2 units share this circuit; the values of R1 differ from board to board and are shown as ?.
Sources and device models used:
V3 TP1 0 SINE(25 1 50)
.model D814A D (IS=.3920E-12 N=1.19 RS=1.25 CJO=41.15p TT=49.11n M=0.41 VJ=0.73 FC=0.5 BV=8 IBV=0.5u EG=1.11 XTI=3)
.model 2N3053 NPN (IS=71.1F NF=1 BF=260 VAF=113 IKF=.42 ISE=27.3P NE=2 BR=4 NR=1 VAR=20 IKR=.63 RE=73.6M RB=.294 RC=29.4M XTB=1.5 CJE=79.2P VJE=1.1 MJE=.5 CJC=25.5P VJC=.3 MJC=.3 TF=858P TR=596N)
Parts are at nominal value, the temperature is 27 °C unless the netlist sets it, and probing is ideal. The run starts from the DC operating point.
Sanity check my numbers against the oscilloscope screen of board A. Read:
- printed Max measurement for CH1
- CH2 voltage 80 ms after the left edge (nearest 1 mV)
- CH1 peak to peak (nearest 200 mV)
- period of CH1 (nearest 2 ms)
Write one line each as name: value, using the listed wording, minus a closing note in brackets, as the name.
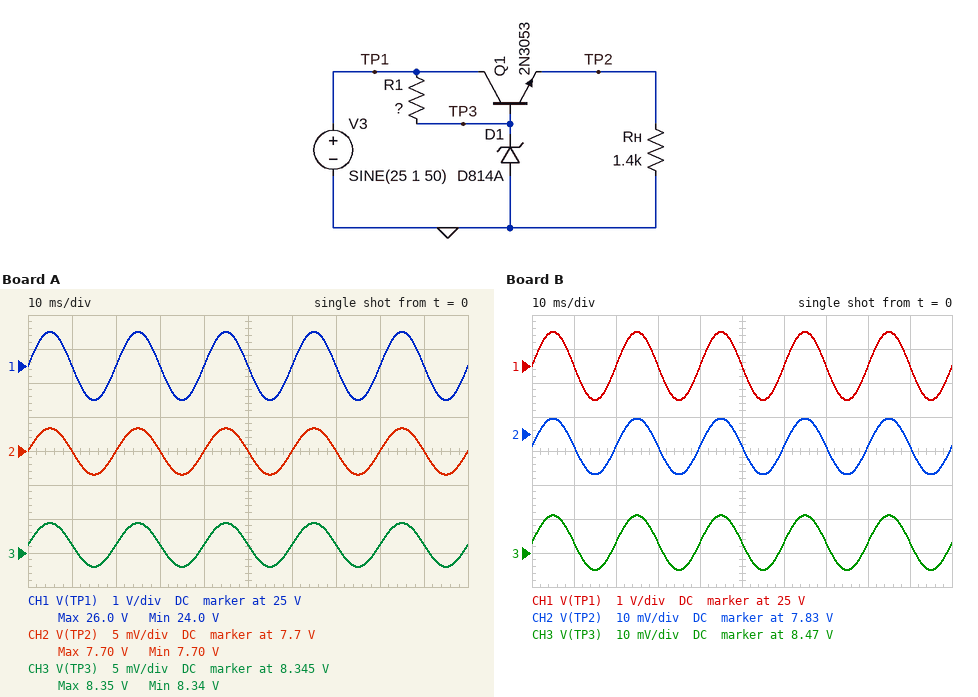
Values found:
printed Max measurement for CH1: 26.0 V
CH2 voltage 80 ms after the left edge: 7.700 V
CH1 peak to peak: 2.0 V
period of CH1: 20 ms
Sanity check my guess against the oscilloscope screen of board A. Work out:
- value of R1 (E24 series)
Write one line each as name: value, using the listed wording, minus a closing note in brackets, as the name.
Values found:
value of R1: 910 Ω
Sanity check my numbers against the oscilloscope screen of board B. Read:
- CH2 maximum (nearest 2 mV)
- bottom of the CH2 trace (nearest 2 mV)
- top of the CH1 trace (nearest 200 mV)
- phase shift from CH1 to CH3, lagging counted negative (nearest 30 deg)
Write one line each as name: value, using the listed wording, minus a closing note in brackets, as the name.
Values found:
CH2 maximum: 7.834 V
bottom of the CH2 trace: 7.818 V
top of the CH1 trace: 26.0 V
phase shift from CH1 to CH3, lagging counted negative: 0 deg
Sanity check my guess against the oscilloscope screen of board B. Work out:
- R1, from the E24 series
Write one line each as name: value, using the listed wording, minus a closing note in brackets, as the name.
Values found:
R1, from the E24 series: 200 Ω
